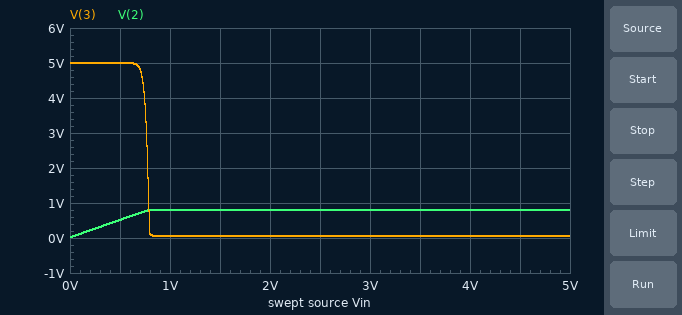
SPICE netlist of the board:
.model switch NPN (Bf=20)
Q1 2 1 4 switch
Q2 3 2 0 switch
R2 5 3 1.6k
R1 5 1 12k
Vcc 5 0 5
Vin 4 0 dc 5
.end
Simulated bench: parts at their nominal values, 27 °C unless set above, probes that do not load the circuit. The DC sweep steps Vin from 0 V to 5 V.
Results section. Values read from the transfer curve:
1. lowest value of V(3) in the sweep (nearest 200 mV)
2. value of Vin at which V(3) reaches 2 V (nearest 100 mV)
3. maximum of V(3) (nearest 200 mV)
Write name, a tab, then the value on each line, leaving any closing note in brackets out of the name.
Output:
lowest value of V(3) in the sweep	0 V
value of Vin at which V(3) reaches 2 V	800 mV
maximum of V(3)	5.0 V
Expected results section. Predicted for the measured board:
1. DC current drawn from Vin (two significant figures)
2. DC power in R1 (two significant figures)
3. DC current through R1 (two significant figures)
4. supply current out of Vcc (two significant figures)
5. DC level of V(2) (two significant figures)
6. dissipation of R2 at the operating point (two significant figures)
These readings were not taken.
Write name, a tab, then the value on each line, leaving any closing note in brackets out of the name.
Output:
DC current drawn from Vin	290 µA
DC power in R1	990 µW
DC current through R1	290 µA
supply current out of Vcc	3.4 mA
DC level of V(2)	810 mV
dissipation of R2 at the operating point	15 mW
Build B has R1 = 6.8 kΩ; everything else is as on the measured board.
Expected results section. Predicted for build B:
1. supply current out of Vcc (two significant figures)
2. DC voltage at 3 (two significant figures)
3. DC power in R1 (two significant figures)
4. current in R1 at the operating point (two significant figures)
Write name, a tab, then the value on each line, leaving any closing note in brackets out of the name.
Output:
supply current out of Vcc	3.6 mA
DC voltage at 3	46 mV
DC power in R1	1.7 mW
current in R1 at the operating point	500 µA
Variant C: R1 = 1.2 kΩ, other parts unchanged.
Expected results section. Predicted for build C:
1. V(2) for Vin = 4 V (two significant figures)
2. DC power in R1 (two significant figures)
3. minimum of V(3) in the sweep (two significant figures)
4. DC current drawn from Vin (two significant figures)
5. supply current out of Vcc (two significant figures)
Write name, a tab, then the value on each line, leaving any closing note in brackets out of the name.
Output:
V(2) for Vin = 4 V	840 mV
DC power in R1	9.4 mW
minimum of V(3) in the sweep	25 mV
DC current drawn from Vin	2.8 mA
supply current out of Vcc	5.9 mA
